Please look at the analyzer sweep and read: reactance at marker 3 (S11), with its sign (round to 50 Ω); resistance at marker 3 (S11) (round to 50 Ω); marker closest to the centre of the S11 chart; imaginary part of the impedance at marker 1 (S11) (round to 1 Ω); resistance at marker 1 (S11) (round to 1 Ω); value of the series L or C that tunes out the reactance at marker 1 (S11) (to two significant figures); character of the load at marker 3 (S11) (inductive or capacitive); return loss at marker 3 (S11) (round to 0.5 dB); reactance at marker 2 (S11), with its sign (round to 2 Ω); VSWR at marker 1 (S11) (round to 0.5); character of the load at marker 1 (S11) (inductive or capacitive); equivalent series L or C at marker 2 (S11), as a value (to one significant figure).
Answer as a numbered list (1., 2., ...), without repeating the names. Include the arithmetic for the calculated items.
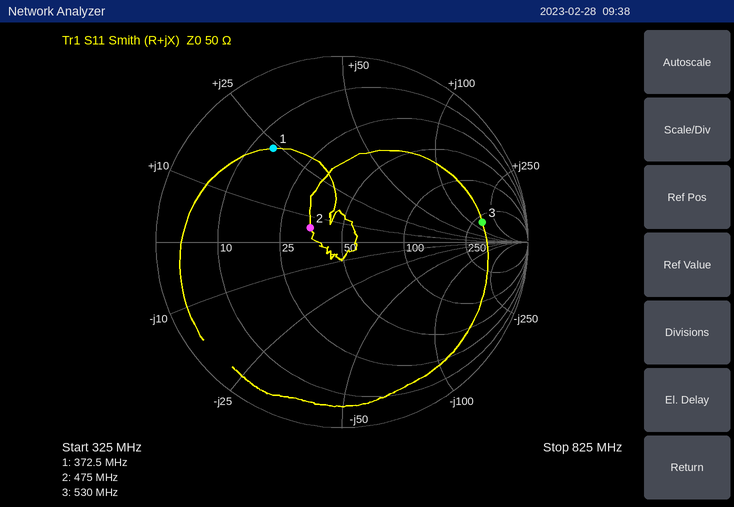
1. +150 Ω
2. 300 Ω
3. marker 2
4. +24 Ω
5. 14 Ω
6. C = 1/(2π × 372.5 MHz × 24 Ω) ≈ 18 pF
7. inductive
8. 2.5 dB
9. +6 Ω
10. 4.5
11. inductive
12. L = 6 Ω/(2π × 475 MHz) ≈ 2 nH
